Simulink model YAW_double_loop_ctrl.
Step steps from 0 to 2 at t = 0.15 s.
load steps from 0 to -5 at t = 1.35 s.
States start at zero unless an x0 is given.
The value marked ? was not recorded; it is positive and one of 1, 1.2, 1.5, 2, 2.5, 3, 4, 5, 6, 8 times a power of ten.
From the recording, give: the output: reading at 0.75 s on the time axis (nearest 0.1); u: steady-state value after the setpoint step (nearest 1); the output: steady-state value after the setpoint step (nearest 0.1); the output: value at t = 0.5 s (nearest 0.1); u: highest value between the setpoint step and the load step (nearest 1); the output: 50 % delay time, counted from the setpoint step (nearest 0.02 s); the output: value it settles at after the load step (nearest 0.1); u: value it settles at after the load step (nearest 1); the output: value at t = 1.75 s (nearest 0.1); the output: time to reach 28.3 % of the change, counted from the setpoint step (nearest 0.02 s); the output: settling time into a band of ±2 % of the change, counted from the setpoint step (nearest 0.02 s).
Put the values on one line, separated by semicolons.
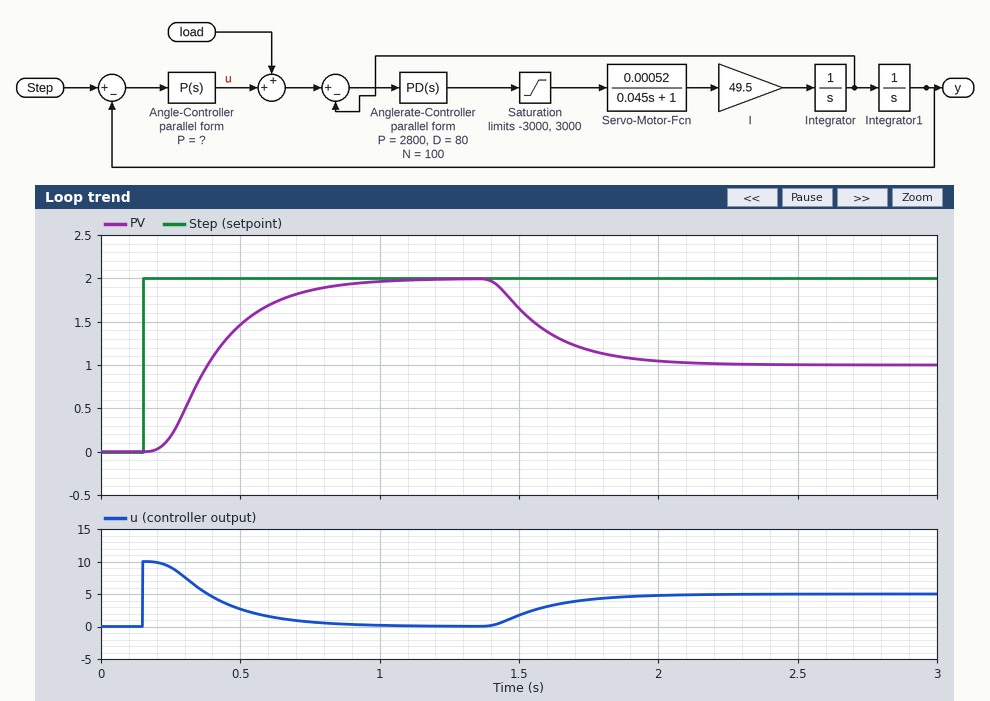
1.9; 0; 2.0; 1.5; 10; 0.24 s; 1.0; 5; 1.2; 0.16 s; 0.84 s
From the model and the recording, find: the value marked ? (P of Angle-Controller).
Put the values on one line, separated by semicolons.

5
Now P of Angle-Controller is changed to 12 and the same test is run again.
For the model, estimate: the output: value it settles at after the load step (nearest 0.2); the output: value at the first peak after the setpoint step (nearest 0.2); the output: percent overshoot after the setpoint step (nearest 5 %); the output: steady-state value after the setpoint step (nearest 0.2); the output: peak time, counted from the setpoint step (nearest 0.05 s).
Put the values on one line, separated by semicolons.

1.6; 2.2; 15 %; 2.0; 0.40 s
